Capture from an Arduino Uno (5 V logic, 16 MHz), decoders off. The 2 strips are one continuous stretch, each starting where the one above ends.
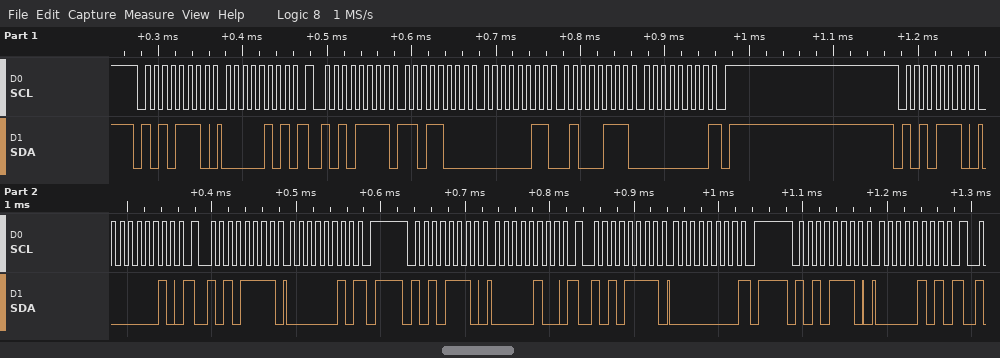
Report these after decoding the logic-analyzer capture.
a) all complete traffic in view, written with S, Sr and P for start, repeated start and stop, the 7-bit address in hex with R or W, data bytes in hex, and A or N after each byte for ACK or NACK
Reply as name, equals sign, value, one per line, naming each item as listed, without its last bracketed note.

all complete traffic in view, written with S, Sr and P for start, repeated start and stop, the 7-bit address in hex with R or W, data bytes in hex, and A or N after each byte for ACK or NACK = S 57W A 05 A Sr 57R A D8 A 03 A 47 A 00 N P S 57W A 02 A Sr 57R A 02 N P S 57W A 04 A Sr 57R A 00 N P S 57W A 05 A
